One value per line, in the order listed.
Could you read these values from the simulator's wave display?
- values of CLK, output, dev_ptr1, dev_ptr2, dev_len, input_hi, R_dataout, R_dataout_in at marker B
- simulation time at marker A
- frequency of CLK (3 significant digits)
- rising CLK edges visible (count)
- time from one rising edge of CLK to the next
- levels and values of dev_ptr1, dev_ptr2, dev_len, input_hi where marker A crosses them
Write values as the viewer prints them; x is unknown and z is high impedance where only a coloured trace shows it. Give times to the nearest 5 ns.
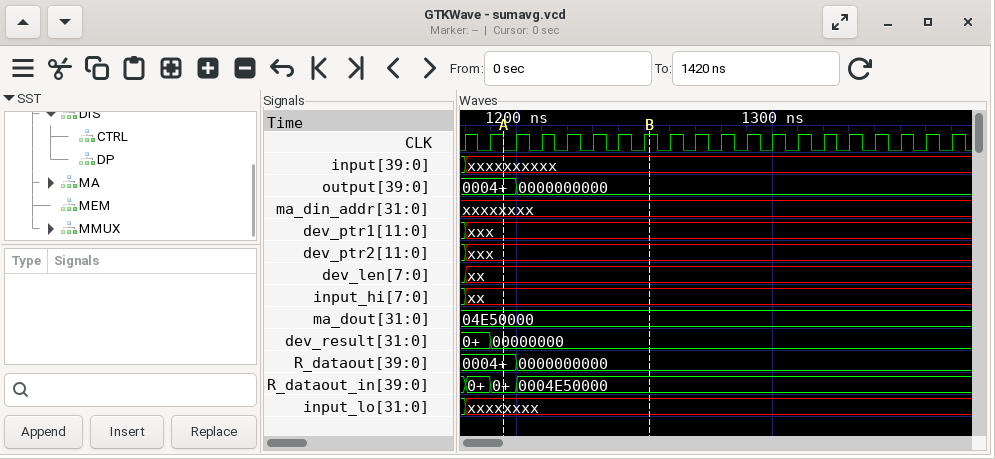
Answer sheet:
CLK=1, output=0000000000, dev_ptr1=xxx, dev_ptr2=xxx, dev_len=xx, input_hi=xx, R_dataout=0000000000, R_dataout_in=0004E50000
1195 ns
100 MHz
20
10 ns
dev_ptr1=xxx, dev_ptr2=xxx, dev_len=xx, input_hi=xx
